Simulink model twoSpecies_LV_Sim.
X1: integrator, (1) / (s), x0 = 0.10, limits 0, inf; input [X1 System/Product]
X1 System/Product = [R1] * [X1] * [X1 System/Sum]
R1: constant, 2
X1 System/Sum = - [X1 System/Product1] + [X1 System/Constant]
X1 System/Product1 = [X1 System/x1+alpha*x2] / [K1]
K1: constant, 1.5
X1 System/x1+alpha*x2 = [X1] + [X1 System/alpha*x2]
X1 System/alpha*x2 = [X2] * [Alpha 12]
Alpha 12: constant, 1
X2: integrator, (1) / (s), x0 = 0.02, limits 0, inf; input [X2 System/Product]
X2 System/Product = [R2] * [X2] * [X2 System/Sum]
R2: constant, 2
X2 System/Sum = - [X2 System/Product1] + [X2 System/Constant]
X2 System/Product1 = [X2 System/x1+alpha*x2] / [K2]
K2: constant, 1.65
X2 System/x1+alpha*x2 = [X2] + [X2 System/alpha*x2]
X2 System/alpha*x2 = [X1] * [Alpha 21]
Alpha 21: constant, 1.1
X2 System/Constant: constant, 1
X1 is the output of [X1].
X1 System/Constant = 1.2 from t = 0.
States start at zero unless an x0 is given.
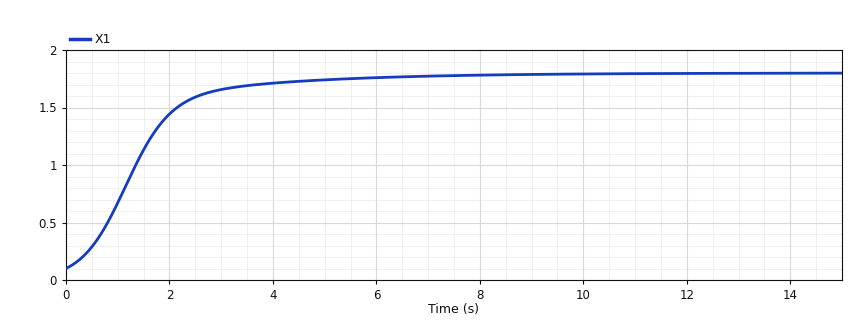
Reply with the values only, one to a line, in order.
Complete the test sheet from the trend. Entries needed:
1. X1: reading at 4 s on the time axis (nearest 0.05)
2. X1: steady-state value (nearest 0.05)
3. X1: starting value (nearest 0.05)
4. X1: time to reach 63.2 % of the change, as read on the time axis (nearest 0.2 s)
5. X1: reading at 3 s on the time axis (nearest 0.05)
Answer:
1.70
1.80
0.10
1.6 s
1.65
